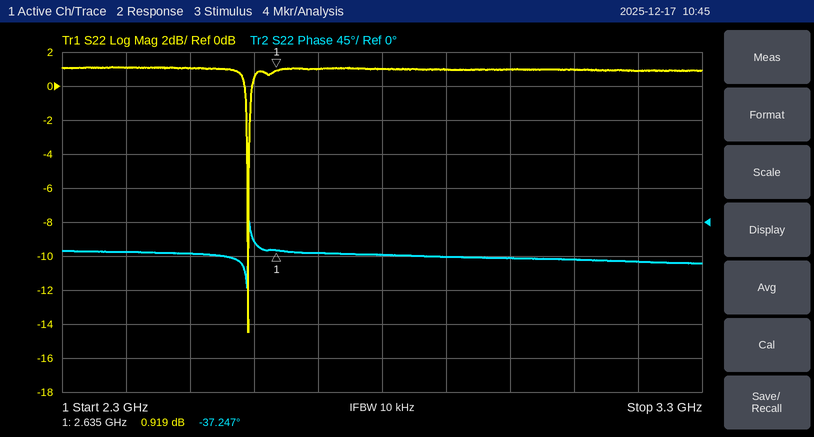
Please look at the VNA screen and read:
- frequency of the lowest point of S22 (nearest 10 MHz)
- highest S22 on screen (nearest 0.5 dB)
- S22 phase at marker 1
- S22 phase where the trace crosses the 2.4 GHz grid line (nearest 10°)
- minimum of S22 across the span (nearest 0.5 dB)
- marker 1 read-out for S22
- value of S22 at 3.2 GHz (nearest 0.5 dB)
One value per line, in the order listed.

2.59 GHz
1.0 dB
-37.247°
-40°
-14.5 dB
0.919 dB
1.0 dB
